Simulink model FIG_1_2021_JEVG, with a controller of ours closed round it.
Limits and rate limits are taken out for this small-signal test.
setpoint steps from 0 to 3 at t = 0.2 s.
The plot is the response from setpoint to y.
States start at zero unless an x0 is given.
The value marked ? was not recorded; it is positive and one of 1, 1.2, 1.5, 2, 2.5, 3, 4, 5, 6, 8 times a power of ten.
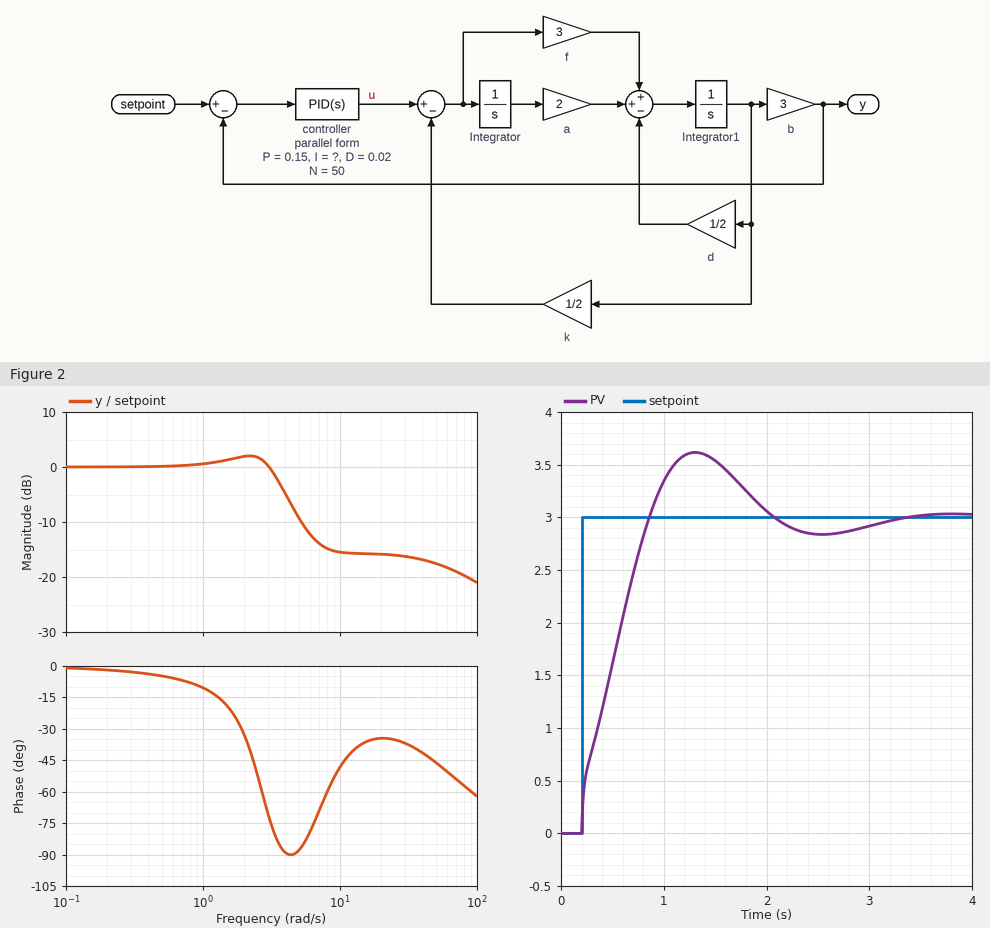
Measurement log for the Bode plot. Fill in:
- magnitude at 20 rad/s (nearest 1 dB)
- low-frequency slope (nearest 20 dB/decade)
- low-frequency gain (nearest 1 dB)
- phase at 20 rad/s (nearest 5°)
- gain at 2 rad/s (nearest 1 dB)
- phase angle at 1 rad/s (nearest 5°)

-16 dB
0 dB/decade
0 dB
-35°
2 dB
-10°
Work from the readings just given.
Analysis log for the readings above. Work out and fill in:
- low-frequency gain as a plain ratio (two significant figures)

1.0
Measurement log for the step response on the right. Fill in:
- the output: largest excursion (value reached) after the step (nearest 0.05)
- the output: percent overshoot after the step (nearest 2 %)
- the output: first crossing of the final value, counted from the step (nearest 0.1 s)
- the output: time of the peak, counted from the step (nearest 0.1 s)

3.60
20 %
0.7 s
1.1 s
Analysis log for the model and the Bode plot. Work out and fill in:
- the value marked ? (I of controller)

1
